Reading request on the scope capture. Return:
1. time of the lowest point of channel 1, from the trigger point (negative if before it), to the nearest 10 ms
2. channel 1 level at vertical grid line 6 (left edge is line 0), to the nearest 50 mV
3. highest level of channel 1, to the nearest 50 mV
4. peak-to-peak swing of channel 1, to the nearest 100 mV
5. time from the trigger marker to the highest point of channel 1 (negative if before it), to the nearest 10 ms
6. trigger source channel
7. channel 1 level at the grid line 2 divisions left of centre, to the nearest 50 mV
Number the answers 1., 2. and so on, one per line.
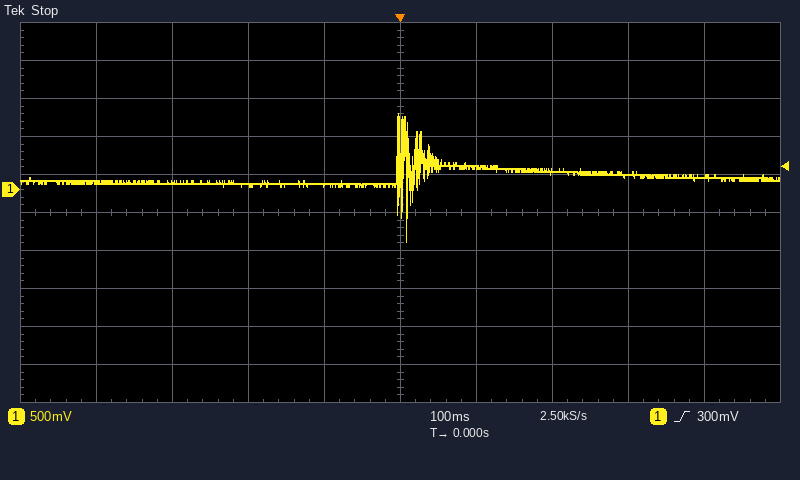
1. +10 ms
2. 300 mV
3. 1.00 V
4. 1.70 V
5. 0 ms
6. channel 1
7. 50 mV
